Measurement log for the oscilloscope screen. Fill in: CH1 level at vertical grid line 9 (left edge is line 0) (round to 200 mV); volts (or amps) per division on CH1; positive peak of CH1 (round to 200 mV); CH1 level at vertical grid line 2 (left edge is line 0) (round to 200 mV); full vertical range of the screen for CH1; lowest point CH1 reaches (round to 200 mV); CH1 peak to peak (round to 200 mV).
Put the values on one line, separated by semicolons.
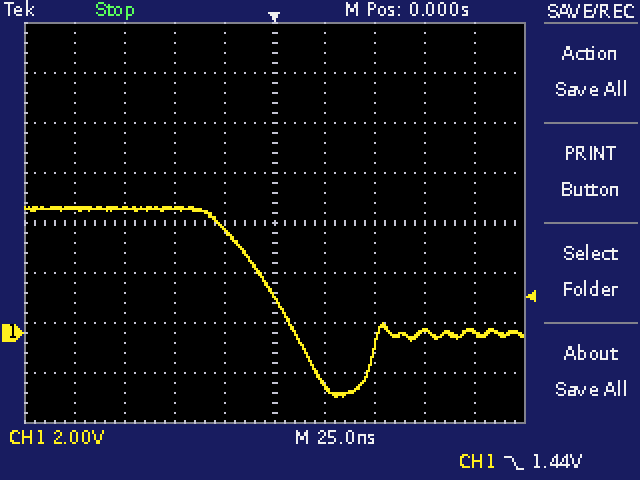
0.0 V; 2 V; 5.0 V; 5.0 V; 16 V; -2.6 V; 7.6 V
